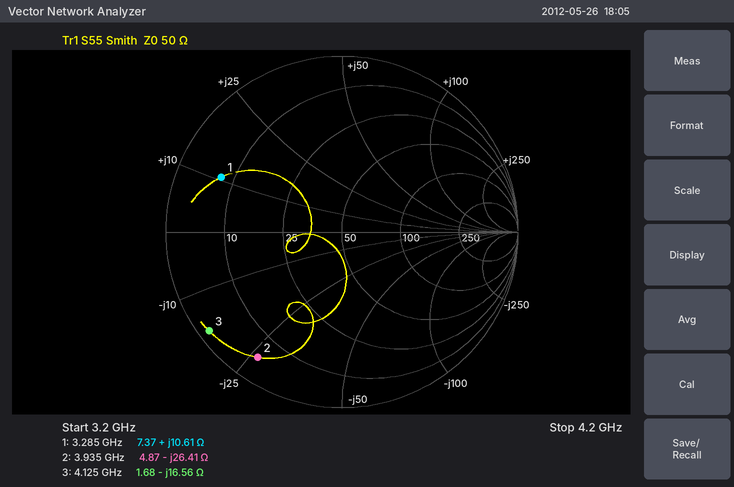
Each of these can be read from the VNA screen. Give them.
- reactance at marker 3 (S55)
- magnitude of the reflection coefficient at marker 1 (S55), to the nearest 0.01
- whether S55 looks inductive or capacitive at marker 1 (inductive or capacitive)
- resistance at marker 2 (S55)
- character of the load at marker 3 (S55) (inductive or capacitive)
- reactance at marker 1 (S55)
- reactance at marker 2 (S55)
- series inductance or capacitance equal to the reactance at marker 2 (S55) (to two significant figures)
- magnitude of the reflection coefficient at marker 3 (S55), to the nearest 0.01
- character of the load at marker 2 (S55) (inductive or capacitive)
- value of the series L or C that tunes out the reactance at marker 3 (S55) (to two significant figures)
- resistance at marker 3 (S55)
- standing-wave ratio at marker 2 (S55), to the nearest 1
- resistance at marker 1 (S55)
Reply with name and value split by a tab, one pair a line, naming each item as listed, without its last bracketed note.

reactance at marker 3	-16.56 Ω
magnitude of the reflection coefficient at marker 1 (S55), to the nearest 0.01	0.75
whether S55 looks inductive or capacitive at marker 1	inductive
resistance at marker 2	4.87 Ω
character of the load at marker 3 (S55)	capacitive
reactance at marker 1	+10.61 Ω
reactance at marker 2	-26.41 Ω
series inductance or capacitance equal to the reactance at marker 2 (S55)	1.5 pF
magnitude of the reflection coefficient at marker 3 (S55), to the nearest 0.01	0.94
character of the load at marker 2 (S55)	capacitive
value of the series L or C that tunes out the reactance at marker 3 (S55)	640 pH
resistance at marker 3	1.68 Ω
standing-wave ratio at marker 2 (S55), to the nearest 1	13
resistance at marker 1	7.37 Ω
